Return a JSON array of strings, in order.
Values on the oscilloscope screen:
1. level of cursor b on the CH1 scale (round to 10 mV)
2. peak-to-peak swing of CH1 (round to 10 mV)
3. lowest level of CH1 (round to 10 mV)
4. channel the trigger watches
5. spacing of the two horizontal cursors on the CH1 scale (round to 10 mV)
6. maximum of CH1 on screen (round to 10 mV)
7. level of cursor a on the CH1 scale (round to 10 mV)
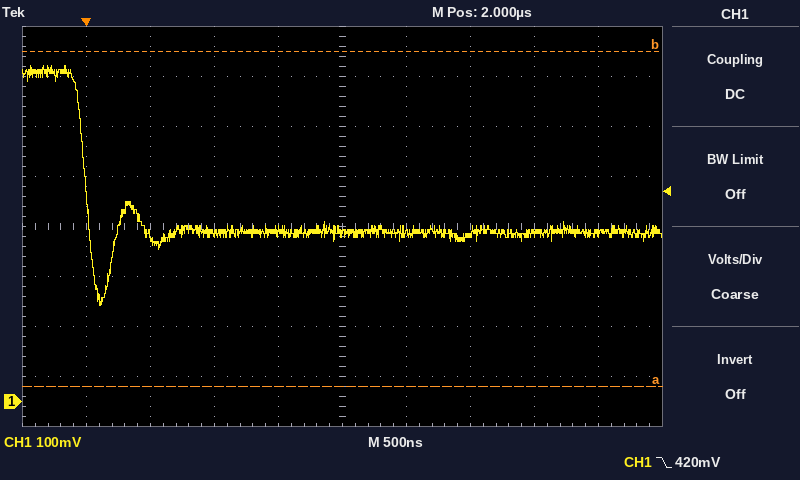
["700 mV", "480 mV", "190 mV", "CH1", "670 mV", "670 mV", "30 mV"]
